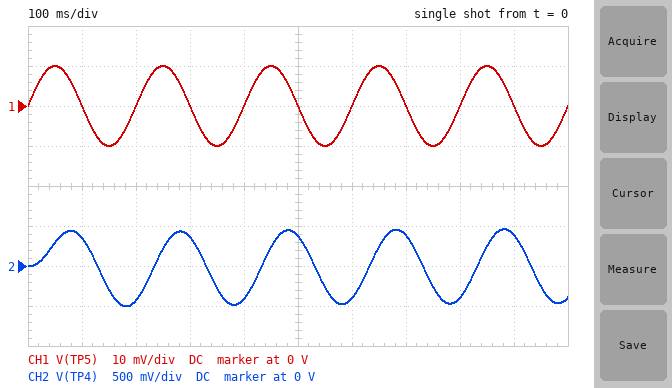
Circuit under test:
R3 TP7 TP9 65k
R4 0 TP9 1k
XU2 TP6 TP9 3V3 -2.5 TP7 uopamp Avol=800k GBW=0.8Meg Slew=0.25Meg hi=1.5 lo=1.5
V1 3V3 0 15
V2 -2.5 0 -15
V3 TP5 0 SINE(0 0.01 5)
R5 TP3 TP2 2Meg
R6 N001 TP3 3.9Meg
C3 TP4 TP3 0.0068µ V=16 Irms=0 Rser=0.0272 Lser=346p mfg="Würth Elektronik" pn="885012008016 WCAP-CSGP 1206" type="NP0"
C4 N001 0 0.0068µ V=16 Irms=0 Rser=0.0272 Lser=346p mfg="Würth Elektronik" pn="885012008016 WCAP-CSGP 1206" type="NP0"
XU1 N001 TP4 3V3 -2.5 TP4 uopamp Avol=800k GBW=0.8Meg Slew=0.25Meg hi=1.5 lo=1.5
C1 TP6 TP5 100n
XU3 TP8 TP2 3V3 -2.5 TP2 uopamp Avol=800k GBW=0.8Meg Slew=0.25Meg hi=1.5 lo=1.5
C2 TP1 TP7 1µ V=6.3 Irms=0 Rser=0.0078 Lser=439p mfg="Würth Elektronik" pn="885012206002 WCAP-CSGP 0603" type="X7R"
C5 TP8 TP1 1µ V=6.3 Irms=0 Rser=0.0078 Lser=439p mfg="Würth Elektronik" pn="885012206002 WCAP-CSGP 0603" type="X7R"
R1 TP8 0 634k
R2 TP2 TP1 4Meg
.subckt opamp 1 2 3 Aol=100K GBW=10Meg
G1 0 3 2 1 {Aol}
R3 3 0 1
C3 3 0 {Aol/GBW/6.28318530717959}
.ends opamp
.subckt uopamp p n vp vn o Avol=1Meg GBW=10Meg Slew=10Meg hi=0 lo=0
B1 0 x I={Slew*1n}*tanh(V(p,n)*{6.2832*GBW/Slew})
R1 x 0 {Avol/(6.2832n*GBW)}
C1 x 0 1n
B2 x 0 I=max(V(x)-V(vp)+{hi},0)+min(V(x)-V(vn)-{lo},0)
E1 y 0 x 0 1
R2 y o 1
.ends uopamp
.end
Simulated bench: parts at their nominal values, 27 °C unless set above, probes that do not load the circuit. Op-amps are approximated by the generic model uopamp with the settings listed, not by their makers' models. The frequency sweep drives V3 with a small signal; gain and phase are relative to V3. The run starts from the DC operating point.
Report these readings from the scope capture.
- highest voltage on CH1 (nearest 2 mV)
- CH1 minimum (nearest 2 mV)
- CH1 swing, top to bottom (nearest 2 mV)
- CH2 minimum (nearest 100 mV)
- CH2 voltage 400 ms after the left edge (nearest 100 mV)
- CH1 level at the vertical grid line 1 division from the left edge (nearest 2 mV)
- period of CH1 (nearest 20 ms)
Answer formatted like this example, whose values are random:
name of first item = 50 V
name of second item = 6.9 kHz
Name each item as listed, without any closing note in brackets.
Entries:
highest voltage on CH1 = 10 mV
CH1 minimum = -10 mV
CH1 swing, top to bottom = 20 mV
CH2 minimum = -500 mV
CH2 voltage 400 ms after the left edge = -400 mV
CH1 level at the vertical grid line 1 division from the left edge = 0 V
period of CH1 = 200 ms
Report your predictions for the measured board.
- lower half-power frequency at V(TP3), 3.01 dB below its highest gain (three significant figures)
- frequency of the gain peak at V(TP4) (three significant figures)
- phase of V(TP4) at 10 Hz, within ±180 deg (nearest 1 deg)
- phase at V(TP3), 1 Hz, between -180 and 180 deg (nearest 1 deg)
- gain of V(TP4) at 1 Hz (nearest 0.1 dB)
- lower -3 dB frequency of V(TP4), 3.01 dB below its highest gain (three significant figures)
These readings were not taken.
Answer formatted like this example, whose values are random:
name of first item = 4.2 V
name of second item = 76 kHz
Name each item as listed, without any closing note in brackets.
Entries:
lower half-power frequency at V(TP3), 3.01 dB below its highest gain = 447 mHz
frequency of the gain peak at V(TP4) = 1.59 Hz
phase of V(TP4) at 10 Hz, within ±180 deg = -97 deg
phase at V(TP3), 1 Hz, between -180 and 180 deg = 22 deg
gain of V(TP4) at 1 Hz = 35.3 dB
lower -3 dB frequency of V(TP4), 3.01 dB below its highest gain = 413 mHz
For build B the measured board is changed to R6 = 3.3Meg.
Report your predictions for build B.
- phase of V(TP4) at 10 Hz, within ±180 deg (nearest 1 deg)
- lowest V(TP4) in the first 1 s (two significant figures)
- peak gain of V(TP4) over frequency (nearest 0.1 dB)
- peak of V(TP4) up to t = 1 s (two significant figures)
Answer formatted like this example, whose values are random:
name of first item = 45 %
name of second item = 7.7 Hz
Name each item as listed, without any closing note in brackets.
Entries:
phase of V(TP4) at 10 Hz, within ±180 deg = -92 deg
lowest V(TP4) in the first 1 s = -540 mV
peak gain of V(TP4) over frequency = 35.7 dB
peak of V(TP4) up to t = 1 s = 490 mV
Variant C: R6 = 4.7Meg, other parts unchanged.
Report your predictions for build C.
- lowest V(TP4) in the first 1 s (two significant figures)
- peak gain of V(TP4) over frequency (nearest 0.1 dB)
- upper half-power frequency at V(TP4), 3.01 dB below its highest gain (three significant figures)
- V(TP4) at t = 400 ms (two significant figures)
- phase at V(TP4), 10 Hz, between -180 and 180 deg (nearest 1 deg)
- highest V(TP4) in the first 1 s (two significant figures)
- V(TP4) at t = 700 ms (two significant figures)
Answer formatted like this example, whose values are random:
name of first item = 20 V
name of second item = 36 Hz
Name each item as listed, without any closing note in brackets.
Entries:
lowest V(TP4) in the first 1 s = -470 mV
peak gain of V(TP4) over frequency = 35.5 dB
upper half-power frequency at V(TP4), 3.01 dB below its highest gain = 5.08 Hz
V(TP4) at t = 400 ms = -400 mV
phase at V(TP4), 10 Hz, between -180 and 180 deg = -101 deg
highest V(TP4) in the first 1 s = 420 mV
V(TP4) at t = 700 ms = 370 mV
